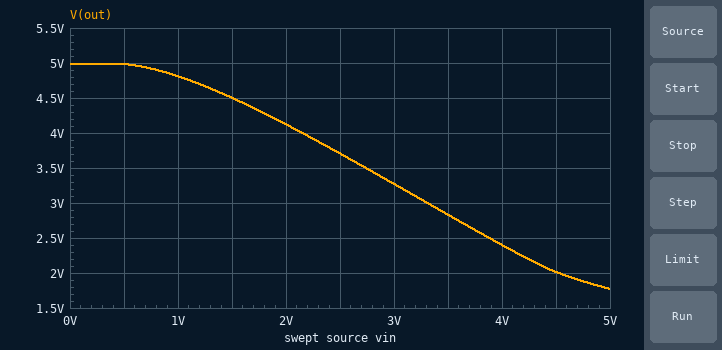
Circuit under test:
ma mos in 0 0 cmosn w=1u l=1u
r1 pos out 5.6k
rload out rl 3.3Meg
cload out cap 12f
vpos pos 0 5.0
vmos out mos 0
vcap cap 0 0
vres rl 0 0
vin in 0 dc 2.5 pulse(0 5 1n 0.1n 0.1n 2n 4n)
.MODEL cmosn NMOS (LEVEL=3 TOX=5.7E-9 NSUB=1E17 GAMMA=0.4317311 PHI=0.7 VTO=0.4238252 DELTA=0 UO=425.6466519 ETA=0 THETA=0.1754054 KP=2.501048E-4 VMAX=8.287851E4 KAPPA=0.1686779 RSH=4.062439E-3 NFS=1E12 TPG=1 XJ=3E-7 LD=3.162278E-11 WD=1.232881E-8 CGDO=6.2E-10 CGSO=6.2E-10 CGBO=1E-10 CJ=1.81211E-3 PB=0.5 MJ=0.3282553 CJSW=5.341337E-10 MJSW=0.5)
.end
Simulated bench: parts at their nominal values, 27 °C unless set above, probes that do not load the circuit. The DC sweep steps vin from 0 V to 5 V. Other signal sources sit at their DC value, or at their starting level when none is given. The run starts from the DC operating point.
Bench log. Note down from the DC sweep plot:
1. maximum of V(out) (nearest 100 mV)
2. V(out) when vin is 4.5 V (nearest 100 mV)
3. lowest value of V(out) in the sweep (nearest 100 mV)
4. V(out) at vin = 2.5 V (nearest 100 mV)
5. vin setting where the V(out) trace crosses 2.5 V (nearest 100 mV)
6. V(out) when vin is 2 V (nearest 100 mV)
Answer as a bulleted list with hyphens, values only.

- 5.0 V
- 2.0 V
- 1.8 V
- 3.7 V
- 3.9 V
- 4.1 V
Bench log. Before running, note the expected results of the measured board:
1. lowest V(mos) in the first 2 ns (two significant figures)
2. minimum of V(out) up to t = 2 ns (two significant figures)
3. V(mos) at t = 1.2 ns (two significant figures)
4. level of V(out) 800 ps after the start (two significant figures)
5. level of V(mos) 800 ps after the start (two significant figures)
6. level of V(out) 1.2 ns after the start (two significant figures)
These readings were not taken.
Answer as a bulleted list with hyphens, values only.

- 1.8 V
- 1.8 V
- 2.0 V
- 5.0 V
- 5.0 V
- 2.0 V
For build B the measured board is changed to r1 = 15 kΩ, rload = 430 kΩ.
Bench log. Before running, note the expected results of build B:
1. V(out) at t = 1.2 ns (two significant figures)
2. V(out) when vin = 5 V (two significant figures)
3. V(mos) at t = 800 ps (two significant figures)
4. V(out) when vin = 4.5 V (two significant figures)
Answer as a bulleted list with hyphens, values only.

- 860 mV
- 590 mV
- 4.8 V
- 650 mV
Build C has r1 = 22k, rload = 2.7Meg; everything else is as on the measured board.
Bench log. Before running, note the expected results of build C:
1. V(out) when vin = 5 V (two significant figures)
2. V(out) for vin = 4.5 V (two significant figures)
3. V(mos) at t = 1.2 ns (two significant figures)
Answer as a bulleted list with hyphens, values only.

- 390 mV
- 430 mV
- 660 mV
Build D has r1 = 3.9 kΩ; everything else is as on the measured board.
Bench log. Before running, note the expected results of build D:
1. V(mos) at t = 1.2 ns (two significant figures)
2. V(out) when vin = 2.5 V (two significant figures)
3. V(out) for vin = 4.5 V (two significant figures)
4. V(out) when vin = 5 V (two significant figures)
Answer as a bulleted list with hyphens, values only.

- 2.7 V
- 4.1 V
- 2.8 V
- 2.5 V
